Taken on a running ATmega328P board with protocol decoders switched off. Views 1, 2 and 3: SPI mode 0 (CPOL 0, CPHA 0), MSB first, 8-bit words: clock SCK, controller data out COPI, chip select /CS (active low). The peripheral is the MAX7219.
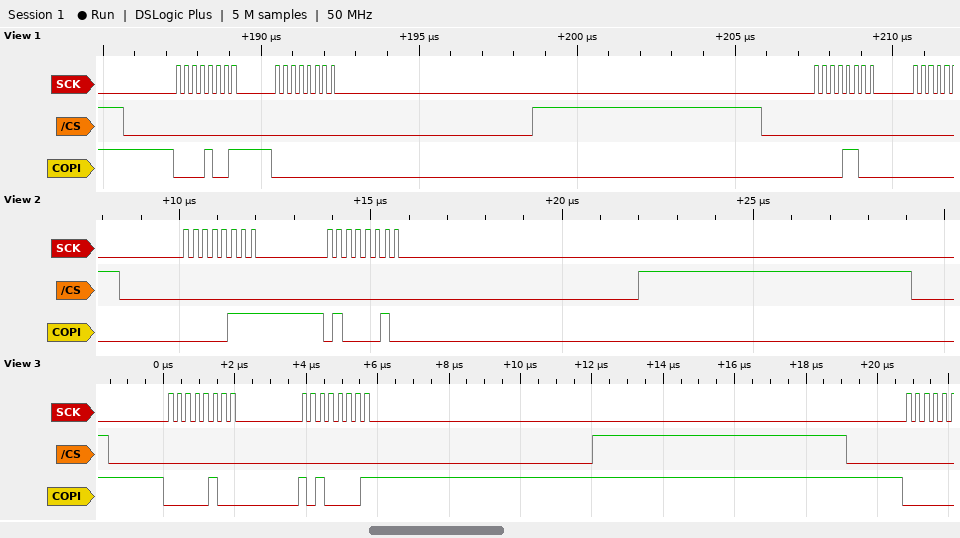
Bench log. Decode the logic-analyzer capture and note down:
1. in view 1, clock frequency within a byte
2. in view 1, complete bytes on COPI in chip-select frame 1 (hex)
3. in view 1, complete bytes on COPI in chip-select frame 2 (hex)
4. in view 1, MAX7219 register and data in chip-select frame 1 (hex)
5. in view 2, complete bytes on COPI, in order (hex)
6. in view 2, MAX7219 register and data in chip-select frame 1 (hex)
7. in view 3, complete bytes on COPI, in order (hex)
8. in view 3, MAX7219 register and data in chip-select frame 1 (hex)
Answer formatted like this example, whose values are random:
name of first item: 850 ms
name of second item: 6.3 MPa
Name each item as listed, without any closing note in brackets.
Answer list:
in view 1, clock frequency within a byte: 4 MHz
in view 1, complete bytes on COPI in chip-select frame 1: 09 00
in view 1, complete bytes on COPI in chip-select frame 2: 0C
in view 1, MAX7219 register and data in chip-select frame 1: register 0x9, data 0x00
in view 2, complete bytes on COPI, in order: 07 42
in view 2, MAX7219 register and data in chip-select frame 1: register 0x7, data 0x42
in view 3, complete bytes on COPI, in order: 04 A1
in view 3, MAX7219 register and data in chip-select frame 1: register 0x4, data 0xA1
